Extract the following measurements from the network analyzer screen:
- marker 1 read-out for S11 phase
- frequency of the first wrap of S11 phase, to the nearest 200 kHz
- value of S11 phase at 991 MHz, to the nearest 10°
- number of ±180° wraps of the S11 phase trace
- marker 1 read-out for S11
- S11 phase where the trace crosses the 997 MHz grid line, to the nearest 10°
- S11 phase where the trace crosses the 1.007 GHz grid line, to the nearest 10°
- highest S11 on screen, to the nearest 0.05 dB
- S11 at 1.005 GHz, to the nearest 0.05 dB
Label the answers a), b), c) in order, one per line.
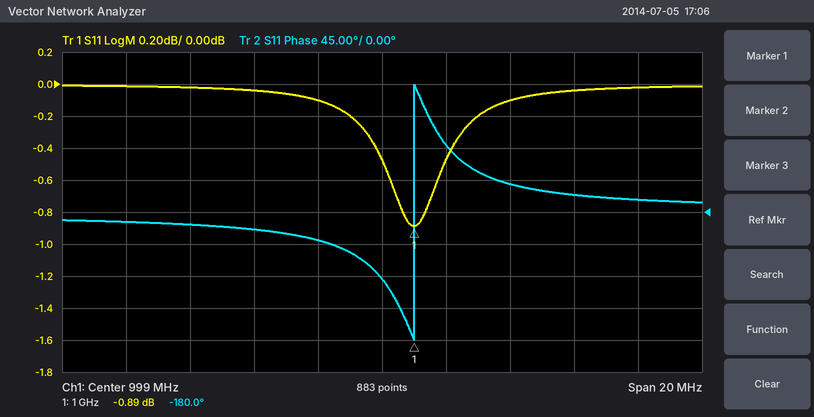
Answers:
a) -180.0°
b) 1.0000 GHz
c) -10°
d) 1
e) -0.89 dB
f) -40°
g) 20°
h) 0.00 dB
i) -0.05 dB
